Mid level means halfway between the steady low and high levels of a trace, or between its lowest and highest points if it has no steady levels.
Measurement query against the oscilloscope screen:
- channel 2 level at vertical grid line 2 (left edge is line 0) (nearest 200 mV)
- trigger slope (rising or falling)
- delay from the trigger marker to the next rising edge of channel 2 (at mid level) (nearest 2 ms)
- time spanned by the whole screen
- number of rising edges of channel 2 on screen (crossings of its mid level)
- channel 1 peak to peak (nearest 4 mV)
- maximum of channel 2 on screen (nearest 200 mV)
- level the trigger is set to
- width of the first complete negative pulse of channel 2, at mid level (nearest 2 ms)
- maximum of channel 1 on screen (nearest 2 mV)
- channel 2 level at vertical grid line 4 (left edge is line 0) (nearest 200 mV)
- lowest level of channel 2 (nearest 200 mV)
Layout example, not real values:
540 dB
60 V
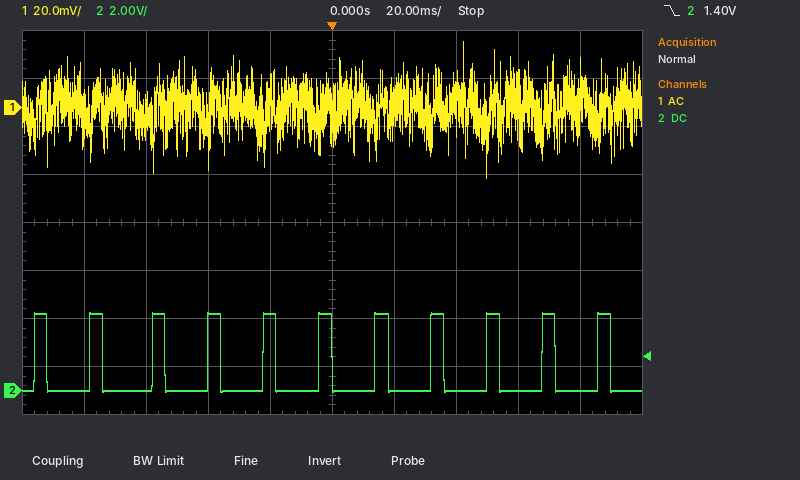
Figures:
0.0 V
falling
14 ms
200 ms
11
56 mV
3.2 V
1.40 V
14 ms
28 mV
3.2 V
0.0 V
